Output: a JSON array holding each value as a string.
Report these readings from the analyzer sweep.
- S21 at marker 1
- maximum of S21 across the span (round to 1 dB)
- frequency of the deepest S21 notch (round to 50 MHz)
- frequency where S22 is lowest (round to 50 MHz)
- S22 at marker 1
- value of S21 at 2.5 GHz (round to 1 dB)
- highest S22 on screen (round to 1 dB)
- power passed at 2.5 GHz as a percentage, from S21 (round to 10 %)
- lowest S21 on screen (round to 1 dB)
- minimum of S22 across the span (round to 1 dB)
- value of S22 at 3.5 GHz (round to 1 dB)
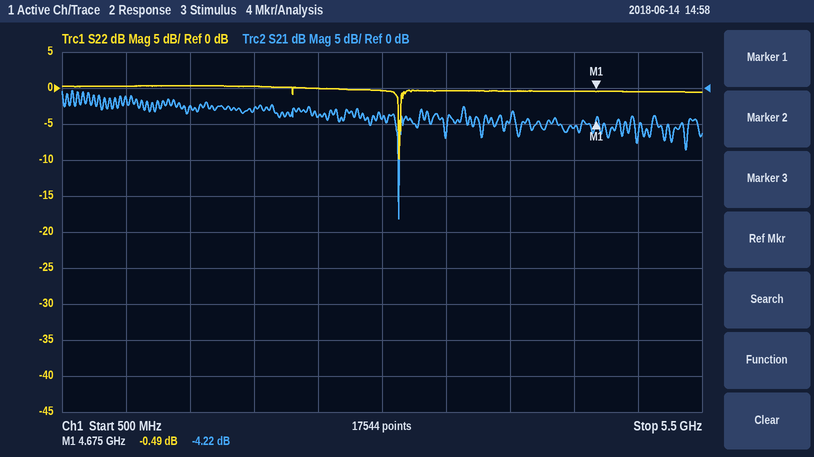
["-4.22 dB", "0 dB", "3.15 GHz", "3.15 GHz", "-0.49 dB", "-4 dB", "0 dB", "40 %", "-18 dB", "-10 dB", "0 dB"]
